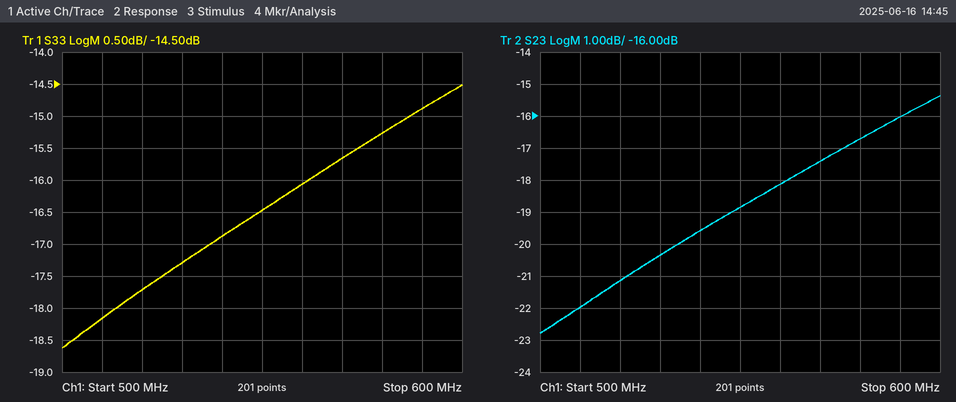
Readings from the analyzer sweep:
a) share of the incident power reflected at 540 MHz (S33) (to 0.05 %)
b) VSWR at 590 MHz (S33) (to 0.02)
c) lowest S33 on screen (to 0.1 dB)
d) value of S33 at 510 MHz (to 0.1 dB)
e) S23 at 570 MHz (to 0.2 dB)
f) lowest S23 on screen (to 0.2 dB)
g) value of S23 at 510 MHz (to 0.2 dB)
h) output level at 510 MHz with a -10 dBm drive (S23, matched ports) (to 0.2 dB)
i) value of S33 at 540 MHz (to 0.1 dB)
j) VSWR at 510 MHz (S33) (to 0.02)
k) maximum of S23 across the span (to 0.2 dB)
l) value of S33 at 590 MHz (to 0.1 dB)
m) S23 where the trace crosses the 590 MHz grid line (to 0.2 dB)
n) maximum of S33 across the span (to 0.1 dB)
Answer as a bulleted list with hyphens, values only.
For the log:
- 2.05 %
- 1.44
- -18.6 dB
- -18.2 dB
- -17.4 dB
- -22.8 dB
- -22.0 dB
- -32.0 dBm
- -16.9 dB
- 1.28
- -15.4 dB
- -14.9 dB
- -16.0 dB
- -14.5 dB
